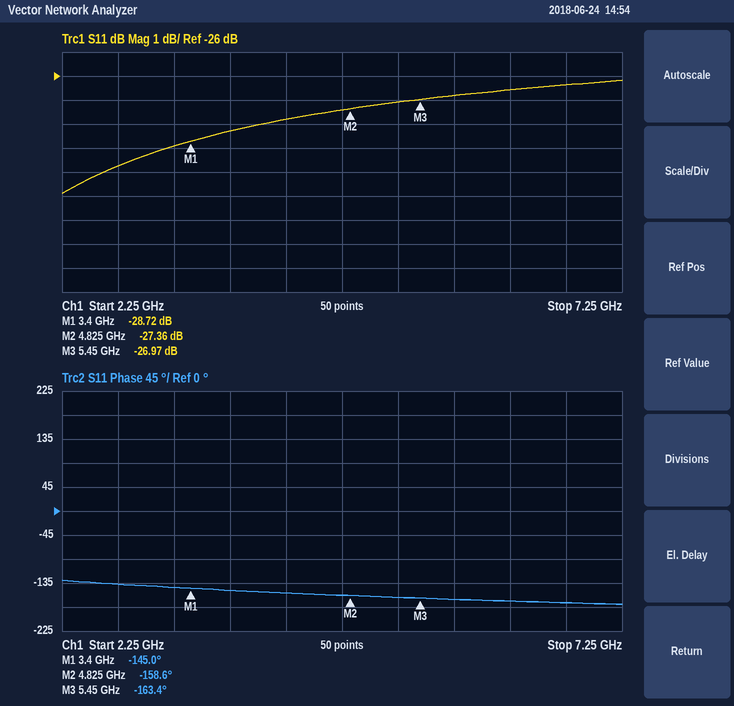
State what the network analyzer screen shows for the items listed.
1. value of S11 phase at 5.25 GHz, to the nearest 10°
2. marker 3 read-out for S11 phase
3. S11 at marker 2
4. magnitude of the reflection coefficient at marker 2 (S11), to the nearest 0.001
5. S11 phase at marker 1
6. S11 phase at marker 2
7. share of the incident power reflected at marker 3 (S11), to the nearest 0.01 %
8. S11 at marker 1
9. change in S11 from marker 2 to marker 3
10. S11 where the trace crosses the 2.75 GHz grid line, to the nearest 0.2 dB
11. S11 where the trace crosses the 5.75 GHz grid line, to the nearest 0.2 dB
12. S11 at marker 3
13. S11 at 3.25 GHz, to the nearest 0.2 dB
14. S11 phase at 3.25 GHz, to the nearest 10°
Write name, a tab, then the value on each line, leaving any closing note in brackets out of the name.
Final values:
value of S11 phase at 5.25 GHz, to the nearest 10°	-160°
marker 3 read-out for S11 phase	-163.4°
S11 at marker 2	-27.36 dB
magnitude of the reflection coefficient at marker 2 (S11), to the nearest 0.001	0.043
S11 phase at marker 1	-145.0°
S11 phase at marker 2	-158.6°
share of the incident power reflected at marker 3 (S11), to the nearest 0.01 %	0.20 %
S11 at marker 1	-28.72 dB
change in S11 from marker 2 to marker 3	0.39 dB
S11 where the trace crosses the 2.75 GHz grid line, to the nearest 0.2 dB	-29.8 dB
S11 where the trace crosses the 5.75 GHz grid line, to the nearest 0.2 dB	-26.8 dB
S11 at marker 3	-26.97 dB
S11 at 3.25 GHz, to the nearest 0.2 dB	-29.0 dB
S11 phase at 3.25 GHz, to the nearest 10°	-140°
